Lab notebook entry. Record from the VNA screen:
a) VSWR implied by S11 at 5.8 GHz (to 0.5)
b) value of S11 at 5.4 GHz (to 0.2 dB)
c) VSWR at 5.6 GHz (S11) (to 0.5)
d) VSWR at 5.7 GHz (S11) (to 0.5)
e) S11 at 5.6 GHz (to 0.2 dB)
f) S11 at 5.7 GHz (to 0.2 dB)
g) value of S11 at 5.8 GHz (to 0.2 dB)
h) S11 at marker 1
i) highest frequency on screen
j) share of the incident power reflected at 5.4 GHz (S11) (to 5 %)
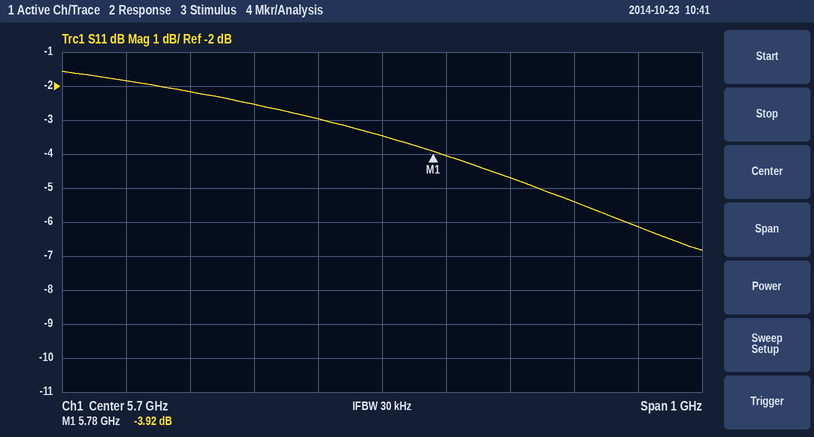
4.5
-2.2 dB
6.0
5.0
-3.0 dB
-3.4 dB
-4.0 dB
-3.92 dB
6.2 GHz
60 %
